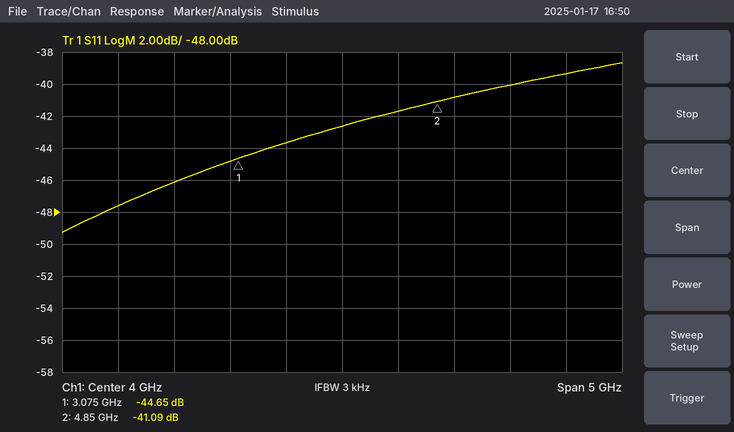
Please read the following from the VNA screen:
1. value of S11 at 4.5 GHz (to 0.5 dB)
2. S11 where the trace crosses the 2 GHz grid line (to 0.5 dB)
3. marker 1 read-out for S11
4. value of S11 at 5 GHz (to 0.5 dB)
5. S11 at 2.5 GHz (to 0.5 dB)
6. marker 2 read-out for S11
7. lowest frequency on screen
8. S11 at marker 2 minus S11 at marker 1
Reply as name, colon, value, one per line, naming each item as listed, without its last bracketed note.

value of S11 at 4.5 GHz: -41.5 dB
S11 where the trace crosses the 2 GHz grid line: -47.5 dB
marker 1 read-out for S11: -44.65 dB
value of S11 at 5 GHz: -41.0 dB
S11 at 2.5 GHz: -46.0 dB
marker 2 read-out for S11: -41.09 dB
lowest frequency on screen: 1.5 GHz
S11 at marker 2 minus S11 at marker 1: 3.56 dB
